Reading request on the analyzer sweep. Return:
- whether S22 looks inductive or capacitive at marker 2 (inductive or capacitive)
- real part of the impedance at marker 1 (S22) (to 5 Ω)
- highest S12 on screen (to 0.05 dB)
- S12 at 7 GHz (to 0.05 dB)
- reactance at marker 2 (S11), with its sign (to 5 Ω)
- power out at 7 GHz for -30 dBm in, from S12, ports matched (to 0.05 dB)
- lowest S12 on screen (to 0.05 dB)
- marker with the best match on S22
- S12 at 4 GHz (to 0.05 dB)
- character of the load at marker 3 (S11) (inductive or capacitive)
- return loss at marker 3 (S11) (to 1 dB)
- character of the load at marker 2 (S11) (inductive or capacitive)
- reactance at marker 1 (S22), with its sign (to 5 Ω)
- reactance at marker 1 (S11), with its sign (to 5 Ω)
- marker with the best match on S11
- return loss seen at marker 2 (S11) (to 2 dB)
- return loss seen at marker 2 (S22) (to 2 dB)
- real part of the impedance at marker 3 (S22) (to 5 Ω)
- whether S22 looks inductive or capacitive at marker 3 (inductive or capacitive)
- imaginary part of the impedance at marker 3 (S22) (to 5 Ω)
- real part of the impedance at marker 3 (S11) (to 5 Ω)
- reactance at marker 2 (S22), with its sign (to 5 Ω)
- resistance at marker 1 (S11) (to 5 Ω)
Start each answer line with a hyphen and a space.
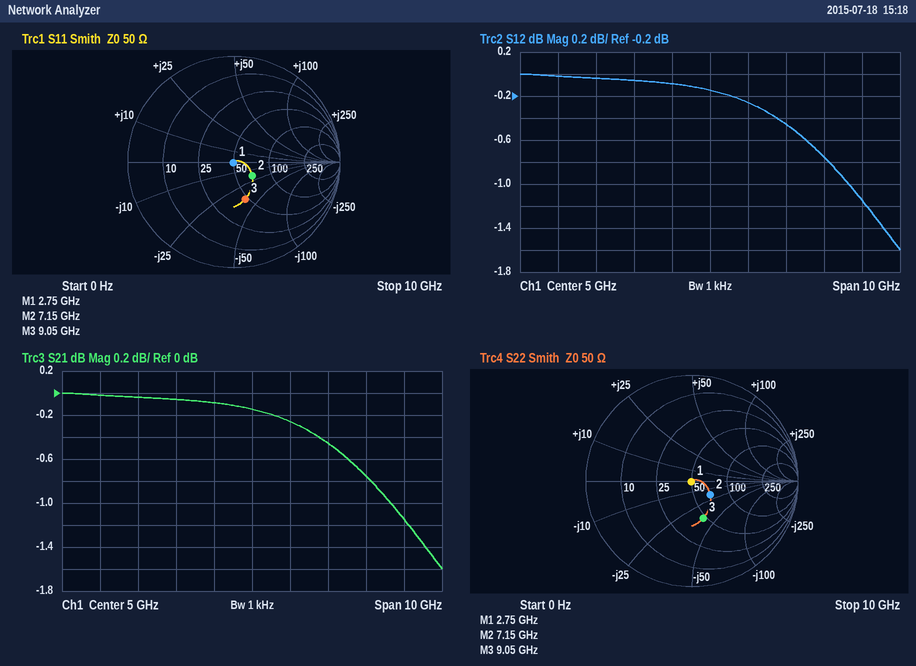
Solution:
- capacitive
- 50 Ω
- 0.00 dB
- -0.45 dB
- -20 Ω
- -30.45 dBm
- -1.60 dB
- marker 1
- -0.10 dB
- capacitive
- 9 dB
- capacitive
- 0 Ω
- 0 Ω
- marker 1
- 14 dB
- 14 dB
- 45 Ω
- capacitive
- -40 Ω
- 45 Ω
- -20 Ω
- 50 Ω
